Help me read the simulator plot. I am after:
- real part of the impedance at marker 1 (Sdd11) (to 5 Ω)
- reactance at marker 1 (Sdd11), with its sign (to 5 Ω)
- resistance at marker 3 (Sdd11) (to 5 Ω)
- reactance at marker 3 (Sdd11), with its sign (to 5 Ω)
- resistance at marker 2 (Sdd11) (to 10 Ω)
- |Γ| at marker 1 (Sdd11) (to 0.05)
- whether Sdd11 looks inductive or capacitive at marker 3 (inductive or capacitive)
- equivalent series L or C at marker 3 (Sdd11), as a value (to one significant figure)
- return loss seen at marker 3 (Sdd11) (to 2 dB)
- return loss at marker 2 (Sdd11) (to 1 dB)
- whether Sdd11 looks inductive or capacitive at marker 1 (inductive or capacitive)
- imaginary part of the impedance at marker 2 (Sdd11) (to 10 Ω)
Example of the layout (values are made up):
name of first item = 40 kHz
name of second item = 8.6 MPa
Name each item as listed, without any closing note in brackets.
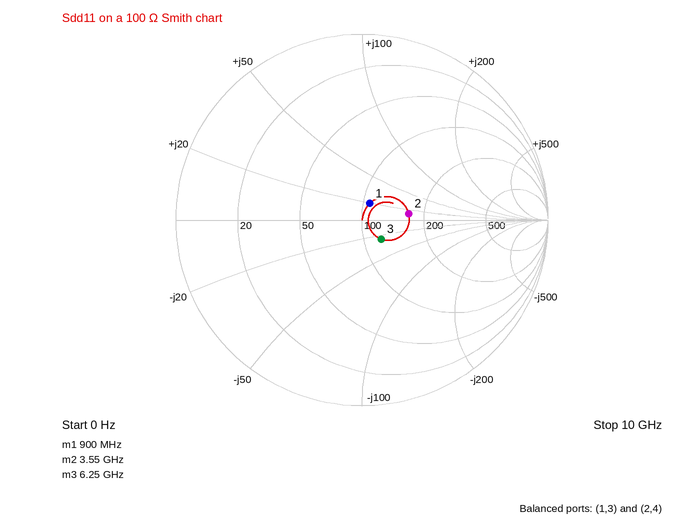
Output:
real part of the impedance at marker 1 (Sdd11) = 105 Ω
reactance at marker 1 (Sdd11), with its sign = +20 Ω
resistance at marker 3 (Sdd11) = 120 Ω
reactance at marker 3 (Sdd11), with its sign = -25 Ω
resistance at marker 2 (Sdd11) = 170 Ω
|Γ| at marker 1 (Sdd11) = 0.10
whether Sdd11 looks inductive or capacitive at marker 3 = capacitive
equivalent series L or C at marker 3 (Sdd11), as a value = 1 pF
return loss seen at marker 3 (Sdd11) = 16 dB
return loss at marker 2 (Sdd11) = 12 dB
whether Sdd11 looks inductive or capacitive at marker 1 = inductive
imaginary part of the impedance at marker 2 (Sdd11) = +10 Ω
